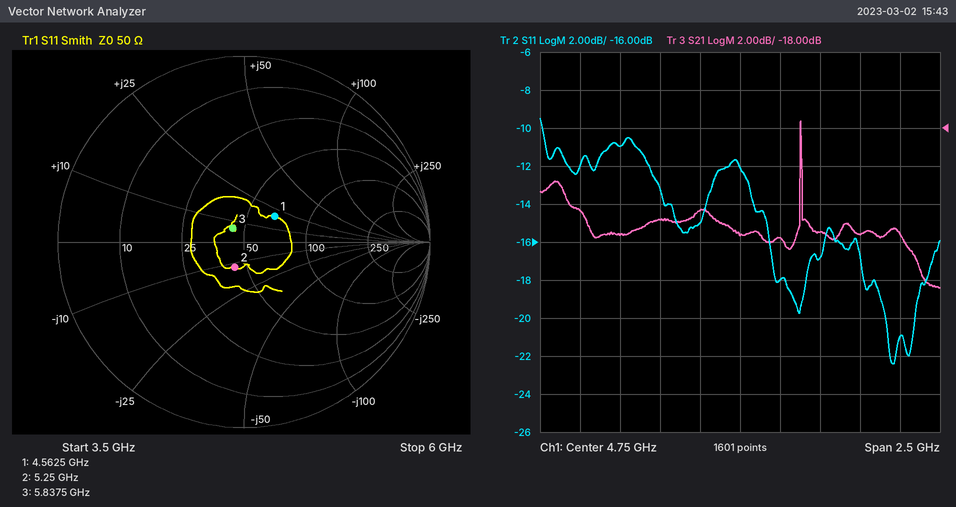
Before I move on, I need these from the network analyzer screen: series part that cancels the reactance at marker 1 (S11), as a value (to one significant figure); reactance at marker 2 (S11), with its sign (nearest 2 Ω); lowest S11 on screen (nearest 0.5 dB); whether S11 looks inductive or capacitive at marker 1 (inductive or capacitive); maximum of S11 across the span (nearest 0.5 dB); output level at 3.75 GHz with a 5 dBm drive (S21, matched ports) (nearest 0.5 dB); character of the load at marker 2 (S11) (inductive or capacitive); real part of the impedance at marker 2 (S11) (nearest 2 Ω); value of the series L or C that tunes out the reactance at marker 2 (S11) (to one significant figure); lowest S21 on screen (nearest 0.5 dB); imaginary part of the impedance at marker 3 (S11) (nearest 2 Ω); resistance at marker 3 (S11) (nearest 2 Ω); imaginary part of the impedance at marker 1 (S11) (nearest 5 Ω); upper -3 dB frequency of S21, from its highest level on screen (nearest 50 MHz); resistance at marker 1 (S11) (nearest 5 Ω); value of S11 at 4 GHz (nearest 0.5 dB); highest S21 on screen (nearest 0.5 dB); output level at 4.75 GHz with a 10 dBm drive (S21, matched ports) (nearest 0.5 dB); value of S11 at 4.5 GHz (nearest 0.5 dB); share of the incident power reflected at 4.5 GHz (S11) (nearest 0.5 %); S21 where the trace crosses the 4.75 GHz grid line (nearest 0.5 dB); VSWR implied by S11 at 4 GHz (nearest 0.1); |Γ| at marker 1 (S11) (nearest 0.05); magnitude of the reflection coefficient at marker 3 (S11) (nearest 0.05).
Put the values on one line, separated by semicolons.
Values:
2 pF; -12 Ω; -22.5 dB; inductive; -9.5 dB; -17.5 dBm; capacitive; 44 Ω; 400 pH; -26.5 dB; +6 Ω; 44 Ω; +20 Ω; 5.15 GHz; 65 Ω; -11.0 dB; -17.5 dB; -13.5 dBm; -15.0 dB; 3.0 %; -23.5 dB; 1.8; 0.20; 0.10
